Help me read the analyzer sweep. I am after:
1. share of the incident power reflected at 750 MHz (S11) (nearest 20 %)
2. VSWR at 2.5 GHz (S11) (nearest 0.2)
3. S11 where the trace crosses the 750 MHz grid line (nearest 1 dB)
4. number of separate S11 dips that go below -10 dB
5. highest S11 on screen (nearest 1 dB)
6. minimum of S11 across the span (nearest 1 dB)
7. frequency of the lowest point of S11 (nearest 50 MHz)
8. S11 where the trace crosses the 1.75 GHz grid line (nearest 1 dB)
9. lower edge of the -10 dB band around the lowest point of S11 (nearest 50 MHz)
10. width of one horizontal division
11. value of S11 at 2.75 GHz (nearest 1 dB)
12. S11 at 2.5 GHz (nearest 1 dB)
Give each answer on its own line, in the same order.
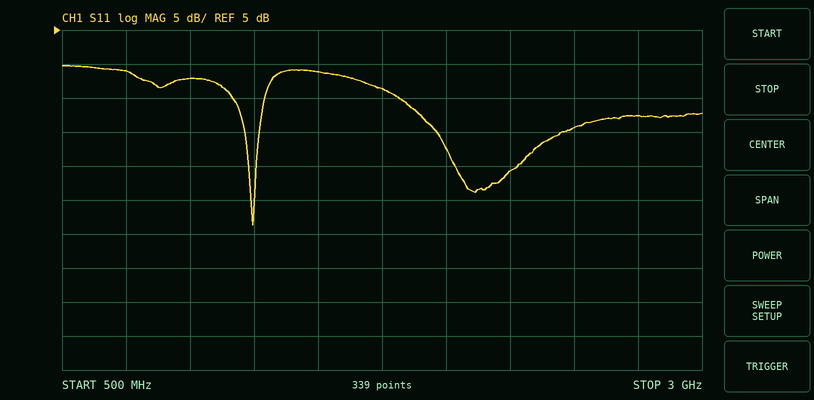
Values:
80 %
2.0
-1 dB
2
0 dB
-24 dB
1.25 GHz
-4 dB
1.20 GHz
250 MHz
-8 dB
-9 dB
